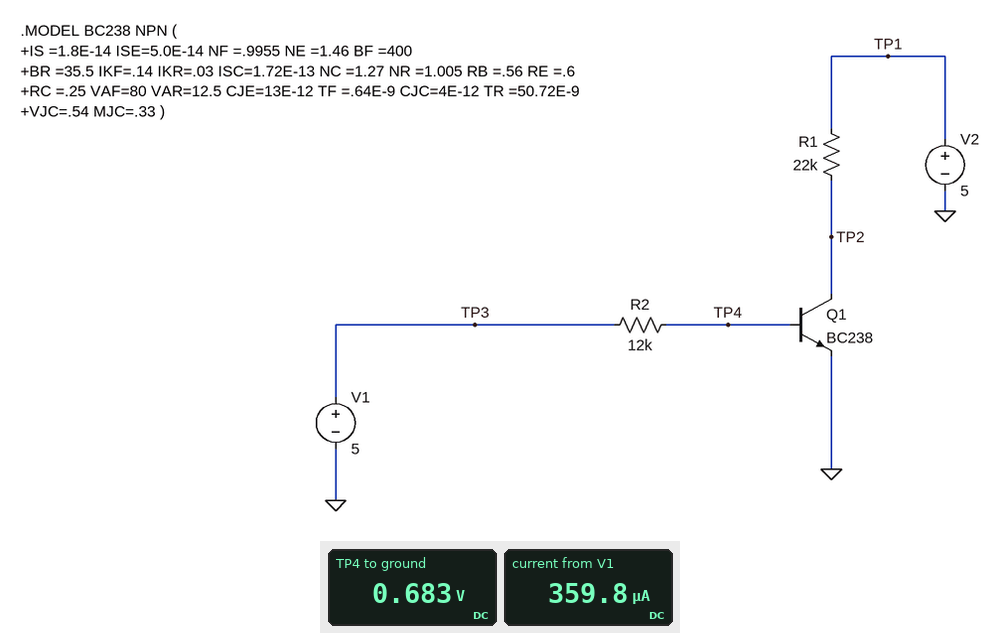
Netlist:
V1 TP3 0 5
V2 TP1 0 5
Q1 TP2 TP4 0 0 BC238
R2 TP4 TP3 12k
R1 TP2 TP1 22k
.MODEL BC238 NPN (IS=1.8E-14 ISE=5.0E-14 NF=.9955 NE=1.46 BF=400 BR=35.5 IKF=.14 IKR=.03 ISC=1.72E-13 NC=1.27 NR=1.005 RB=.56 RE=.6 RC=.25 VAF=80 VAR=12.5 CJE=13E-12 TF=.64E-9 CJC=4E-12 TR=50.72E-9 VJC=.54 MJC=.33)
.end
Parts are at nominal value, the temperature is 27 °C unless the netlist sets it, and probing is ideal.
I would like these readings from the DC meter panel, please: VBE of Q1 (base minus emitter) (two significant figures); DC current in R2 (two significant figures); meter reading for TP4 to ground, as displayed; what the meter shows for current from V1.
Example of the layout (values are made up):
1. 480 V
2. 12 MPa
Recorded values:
1. 680 mV
2. 360 µA
3. 0.683 V
4. 359.8 µA
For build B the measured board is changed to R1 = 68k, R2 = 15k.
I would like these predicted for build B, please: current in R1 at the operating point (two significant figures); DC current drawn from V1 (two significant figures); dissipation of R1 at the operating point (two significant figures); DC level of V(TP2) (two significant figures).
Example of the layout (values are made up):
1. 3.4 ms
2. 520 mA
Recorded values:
1. 74 µA
2. 290 µA
3. 370 µW
4. -3.6 mV
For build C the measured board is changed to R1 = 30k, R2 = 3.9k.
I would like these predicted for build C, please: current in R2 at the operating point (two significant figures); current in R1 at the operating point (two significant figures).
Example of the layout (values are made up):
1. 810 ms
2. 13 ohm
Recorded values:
1. 1.1 mA
2. 170 µA
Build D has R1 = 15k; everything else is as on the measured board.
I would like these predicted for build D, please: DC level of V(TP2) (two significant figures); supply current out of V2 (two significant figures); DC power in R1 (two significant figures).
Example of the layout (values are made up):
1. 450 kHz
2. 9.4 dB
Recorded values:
1. -2.0 mV
2. 330 µA
3. 1.7 mW
